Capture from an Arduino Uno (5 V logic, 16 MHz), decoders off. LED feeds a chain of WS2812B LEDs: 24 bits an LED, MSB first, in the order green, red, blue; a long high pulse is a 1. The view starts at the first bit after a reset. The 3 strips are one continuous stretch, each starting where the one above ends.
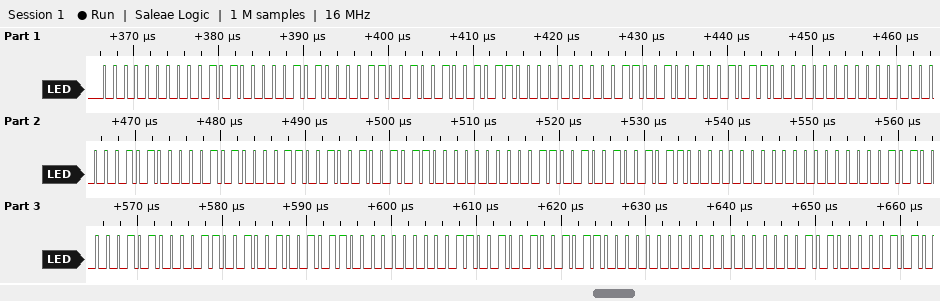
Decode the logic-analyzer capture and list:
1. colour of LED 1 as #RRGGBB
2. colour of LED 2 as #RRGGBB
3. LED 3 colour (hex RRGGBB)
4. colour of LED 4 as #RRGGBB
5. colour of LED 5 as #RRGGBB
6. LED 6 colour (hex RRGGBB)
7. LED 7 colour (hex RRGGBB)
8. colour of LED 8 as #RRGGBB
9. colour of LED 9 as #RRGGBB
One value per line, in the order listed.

#280028
#966400
#966400
#280028
#966400
#966400
#280028
#966400
#966400
